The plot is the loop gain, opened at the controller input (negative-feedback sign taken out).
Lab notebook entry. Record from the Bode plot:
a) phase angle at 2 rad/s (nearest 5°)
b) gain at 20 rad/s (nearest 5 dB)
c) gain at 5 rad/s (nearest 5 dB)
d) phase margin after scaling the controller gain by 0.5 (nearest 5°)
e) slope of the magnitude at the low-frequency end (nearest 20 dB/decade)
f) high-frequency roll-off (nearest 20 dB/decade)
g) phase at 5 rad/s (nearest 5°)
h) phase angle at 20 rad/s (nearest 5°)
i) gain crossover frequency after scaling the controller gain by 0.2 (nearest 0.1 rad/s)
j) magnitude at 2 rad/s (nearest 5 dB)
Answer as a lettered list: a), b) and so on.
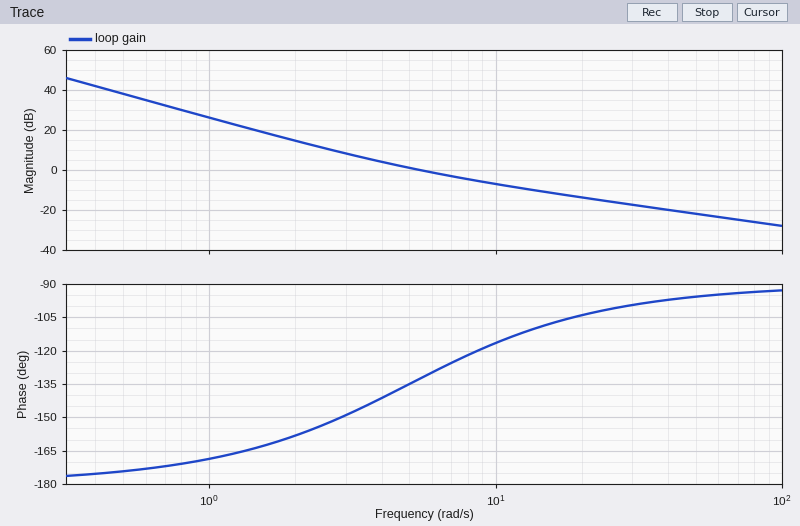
a) -160°
b) -15 dB
c) 0 dB
d) 35°
e) -40 dB/decade
f) -20 dB/decade
g) -135°
h) -105°
i) 2.1 rad/s
j) 15 dB
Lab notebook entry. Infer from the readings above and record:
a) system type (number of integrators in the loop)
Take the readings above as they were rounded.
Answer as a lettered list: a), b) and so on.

a) 2
